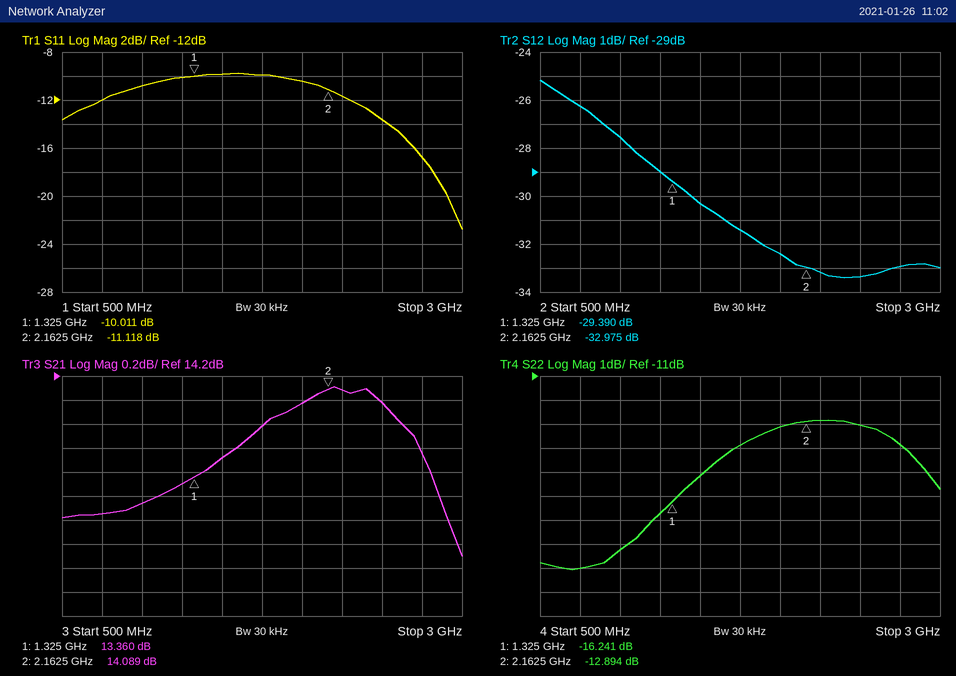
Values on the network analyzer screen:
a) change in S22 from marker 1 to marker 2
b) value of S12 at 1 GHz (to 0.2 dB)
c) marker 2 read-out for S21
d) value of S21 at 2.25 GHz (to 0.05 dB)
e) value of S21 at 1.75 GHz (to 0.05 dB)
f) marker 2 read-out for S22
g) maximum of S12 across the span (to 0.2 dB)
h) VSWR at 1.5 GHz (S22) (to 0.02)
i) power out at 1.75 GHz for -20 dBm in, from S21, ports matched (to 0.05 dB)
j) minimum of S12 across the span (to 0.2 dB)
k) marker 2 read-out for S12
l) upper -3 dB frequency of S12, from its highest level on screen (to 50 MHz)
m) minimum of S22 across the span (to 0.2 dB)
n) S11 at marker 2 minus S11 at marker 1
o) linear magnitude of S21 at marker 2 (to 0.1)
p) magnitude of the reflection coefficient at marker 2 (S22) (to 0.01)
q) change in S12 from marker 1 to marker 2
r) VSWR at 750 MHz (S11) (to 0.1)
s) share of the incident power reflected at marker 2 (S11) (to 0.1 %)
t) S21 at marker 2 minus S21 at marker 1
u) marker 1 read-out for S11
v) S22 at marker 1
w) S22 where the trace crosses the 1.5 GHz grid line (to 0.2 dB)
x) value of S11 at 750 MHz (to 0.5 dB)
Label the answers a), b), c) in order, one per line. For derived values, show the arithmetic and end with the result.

a) -12.894 − (-16.241) = 3.347 dB
b) -27.6 dB
c) 14.089 dB
d) 14.10 dB
e) 13.80 dB
f) -12.894 dB
g) -25.2 dB
h) |Γ| = 10^(-15.2/20) = 0.1738; VSWR = (1 + 0.1738)/(1 − 0.1738) ≈ 1.42
i) -20 dBm + (13.80 dB) = -6.20 dBm
j) -33.4 dB
k) -32.975 dB
l) 1.10 GHz
m) -19.0 dB
n) -11.118 − (-10.011) = -1.107 dB
o) 10^(14.089/20) ≈ 5.1
p) 10^(-12.894/20) ≈ 0.23
q) -32.975 − (-29.39) = -3.585 dB
r) |Γ| = 10^(-12/20) = 0.2512; VSWR = (1 + 0.2512)/(1 − 0.2512) ≈ 1.7
s) 10^(-11.118/10) ≈ 7.7 %
t) 14.089 − (13.36) = 0.729 dB
u) -10.011 dB
v) -16.241 dB
w) -15.2 dB
x) -12.0 dB
